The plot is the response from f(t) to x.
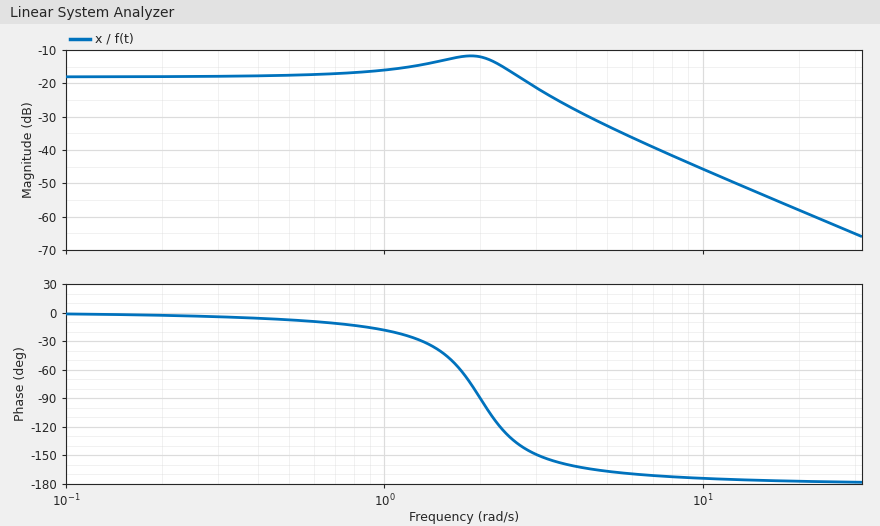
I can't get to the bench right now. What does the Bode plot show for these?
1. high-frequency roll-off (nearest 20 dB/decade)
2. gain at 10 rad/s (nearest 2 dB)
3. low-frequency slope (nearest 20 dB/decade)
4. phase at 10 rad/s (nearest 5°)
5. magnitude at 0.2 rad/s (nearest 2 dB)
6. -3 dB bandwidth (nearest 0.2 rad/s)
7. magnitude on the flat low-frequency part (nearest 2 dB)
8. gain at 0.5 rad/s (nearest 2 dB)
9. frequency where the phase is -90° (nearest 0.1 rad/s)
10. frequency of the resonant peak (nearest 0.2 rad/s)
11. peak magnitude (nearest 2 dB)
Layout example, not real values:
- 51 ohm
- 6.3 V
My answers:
- -40 dB/decade
- -46 dB
- 0 dB/decade
- -175°
- -18 dB
- 3.0 rad/s
- -18 dB
- -18 dB
- 2.0 rad/s
- 1.8 rad/s
- -12 dB
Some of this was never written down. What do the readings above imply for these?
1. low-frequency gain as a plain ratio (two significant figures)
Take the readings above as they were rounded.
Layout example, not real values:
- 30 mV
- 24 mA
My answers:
- 0.13
